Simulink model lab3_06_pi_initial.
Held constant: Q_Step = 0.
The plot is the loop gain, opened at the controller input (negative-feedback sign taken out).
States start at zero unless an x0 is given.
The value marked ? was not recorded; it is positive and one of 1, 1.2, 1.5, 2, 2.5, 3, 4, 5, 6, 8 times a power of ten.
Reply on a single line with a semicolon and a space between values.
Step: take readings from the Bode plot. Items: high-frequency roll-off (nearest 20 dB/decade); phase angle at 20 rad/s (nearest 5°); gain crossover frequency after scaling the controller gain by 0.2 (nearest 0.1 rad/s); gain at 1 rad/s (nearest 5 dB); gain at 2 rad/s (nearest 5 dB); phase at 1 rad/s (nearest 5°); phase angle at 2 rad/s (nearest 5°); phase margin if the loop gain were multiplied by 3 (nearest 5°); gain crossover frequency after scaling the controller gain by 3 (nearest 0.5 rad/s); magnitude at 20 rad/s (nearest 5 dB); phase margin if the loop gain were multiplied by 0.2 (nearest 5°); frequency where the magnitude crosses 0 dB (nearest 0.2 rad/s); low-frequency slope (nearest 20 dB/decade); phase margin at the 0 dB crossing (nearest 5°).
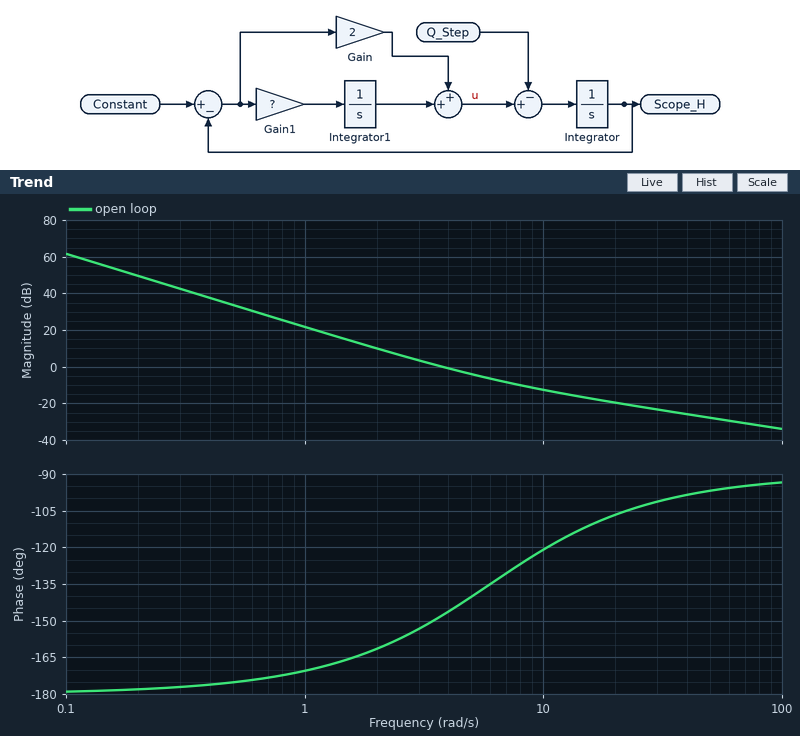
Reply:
-20 dB/decade; -105°; 1.6 rad/s; 20 dB; 10 dB; -170°; -160°; 50°; 7.5 rad/s; -20 dB; 15°; 3.8 rad/s; -40 dB/decade; 30°
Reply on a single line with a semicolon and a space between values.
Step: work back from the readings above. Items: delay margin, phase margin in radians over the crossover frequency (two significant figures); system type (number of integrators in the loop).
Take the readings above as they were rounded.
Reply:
0.14 s; 2
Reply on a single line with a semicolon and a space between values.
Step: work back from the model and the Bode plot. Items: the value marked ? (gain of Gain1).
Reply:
12
